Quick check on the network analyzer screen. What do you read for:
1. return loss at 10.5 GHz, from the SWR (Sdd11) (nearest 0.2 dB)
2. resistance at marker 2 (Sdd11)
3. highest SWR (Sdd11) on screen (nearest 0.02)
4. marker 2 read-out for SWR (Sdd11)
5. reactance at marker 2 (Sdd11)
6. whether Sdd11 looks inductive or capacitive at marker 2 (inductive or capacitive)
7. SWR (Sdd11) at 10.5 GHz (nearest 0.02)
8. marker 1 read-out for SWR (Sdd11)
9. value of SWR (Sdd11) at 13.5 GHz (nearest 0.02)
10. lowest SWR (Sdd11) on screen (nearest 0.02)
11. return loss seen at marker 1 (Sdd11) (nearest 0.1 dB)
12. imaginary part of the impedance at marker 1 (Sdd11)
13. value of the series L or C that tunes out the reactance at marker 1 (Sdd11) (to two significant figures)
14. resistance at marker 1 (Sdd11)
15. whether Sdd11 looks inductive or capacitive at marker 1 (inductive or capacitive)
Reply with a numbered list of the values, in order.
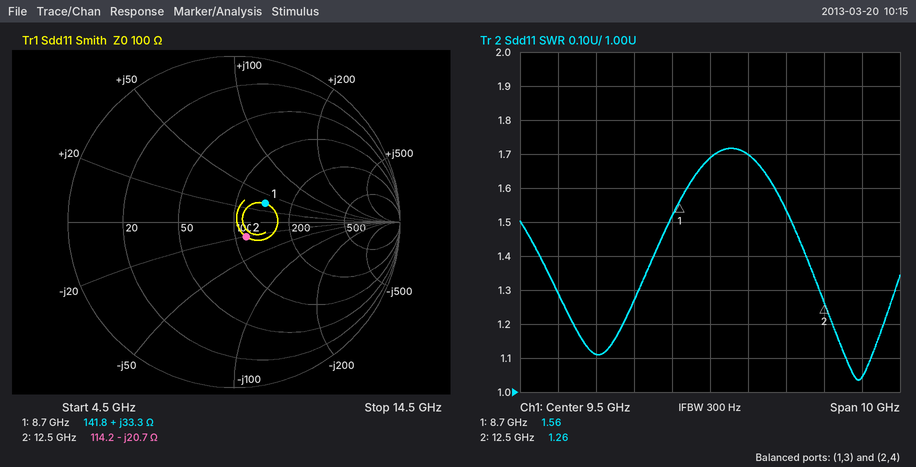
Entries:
1. 11.8 dB
2. 114.2 Ω
3. 1.72
4. 1.26
5. -20.7 Ω
6. capacitive
7. 1.70
8. 1.56
9. 1.04
10. 1.04
11. 13.2 dB
12. +33.3 Ω
13. 550 fF
14. 141.8 Ω
15. inductive
